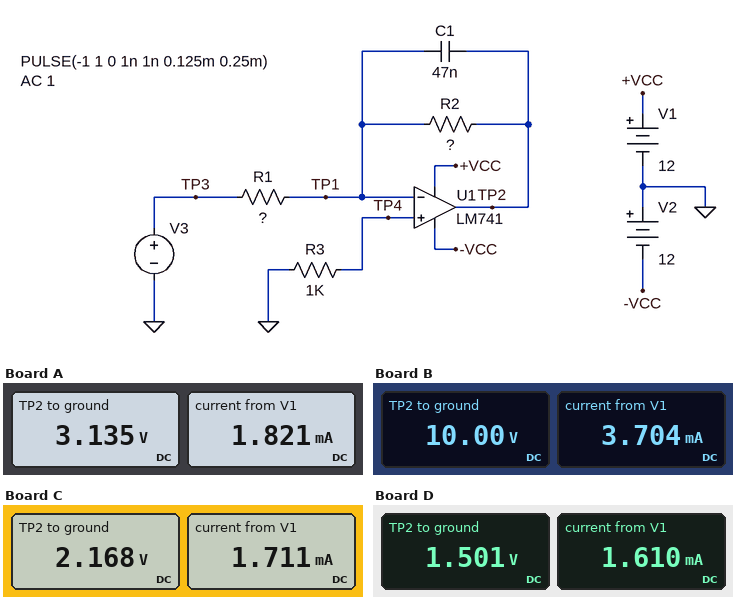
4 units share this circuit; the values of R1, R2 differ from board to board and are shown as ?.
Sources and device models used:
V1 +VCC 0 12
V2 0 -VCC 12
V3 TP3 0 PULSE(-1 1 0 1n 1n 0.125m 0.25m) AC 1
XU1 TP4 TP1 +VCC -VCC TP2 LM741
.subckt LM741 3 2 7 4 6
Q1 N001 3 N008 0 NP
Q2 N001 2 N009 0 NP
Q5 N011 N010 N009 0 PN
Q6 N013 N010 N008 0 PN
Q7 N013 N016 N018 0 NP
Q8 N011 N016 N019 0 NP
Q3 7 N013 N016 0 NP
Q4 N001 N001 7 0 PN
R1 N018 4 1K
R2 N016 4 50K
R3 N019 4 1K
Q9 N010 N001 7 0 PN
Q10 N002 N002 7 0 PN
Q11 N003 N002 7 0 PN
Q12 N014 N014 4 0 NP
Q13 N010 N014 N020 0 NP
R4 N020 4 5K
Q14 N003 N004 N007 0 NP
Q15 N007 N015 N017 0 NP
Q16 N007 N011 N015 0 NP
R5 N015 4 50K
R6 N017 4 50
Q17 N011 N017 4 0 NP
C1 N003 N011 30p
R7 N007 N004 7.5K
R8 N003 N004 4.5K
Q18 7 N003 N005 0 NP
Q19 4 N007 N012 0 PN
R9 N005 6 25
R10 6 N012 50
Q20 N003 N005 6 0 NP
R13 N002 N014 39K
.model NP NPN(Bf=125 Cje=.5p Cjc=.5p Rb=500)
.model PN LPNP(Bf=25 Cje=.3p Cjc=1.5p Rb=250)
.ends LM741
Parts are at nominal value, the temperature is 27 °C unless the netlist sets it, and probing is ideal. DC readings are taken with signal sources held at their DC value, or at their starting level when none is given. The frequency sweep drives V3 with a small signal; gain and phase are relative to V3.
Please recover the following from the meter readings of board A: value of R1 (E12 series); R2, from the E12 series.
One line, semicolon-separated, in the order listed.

1.5 kΩ; 4.7 kΩ
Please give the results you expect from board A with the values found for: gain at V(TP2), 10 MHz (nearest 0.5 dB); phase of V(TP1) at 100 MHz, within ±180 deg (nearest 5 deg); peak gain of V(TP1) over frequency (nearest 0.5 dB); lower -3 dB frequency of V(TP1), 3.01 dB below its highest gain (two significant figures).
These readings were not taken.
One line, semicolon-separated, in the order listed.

-27.0 dB; 10 deg; -22.5 dB; 190 MHz
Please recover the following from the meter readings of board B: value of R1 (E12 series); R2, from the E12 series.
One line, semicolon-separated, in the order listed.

390 Ω; 3.9 kΩ
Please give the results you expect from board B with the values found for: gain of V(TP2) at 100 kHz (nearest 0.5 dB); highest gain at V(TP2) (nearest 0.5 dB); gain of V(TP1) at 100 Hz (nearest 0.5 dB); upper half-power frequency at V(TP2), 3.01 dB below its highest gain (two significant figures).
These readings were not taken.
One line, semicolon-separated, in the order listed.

-20.5 dB; 20.0 dB; -59.5 dB; 860 Hz
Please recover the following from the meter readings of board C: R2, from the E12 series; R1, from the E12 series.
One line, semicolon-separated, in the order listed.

3.9 kΩ; 1.8 kΩ
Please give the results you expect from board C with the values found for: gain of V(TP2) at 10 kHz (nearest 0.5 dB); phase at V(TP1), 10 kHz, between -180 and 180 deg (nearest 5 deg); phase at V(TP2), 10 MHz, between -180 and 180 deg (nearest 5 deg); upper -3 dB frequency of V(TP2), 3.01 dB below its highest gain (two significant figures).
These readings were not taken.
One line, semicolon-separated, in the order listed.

-14.5 dB; 15 deg; 5 deg; 870 Hz
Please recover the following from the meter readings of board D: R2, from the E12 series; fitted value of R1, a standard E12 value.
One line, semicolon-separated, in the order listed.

3.3 kΩ; 2.2 kΩ
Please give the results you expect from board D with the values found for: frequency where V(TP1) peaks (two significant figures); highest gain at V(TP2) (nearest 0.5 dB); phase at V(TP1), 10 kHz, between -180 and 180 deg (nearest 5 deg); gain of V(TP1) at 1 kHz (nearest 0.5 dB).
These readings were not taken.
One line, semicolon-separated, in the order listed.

790 MHz; 3.5 dB; 20 deg; -58.5 dB
